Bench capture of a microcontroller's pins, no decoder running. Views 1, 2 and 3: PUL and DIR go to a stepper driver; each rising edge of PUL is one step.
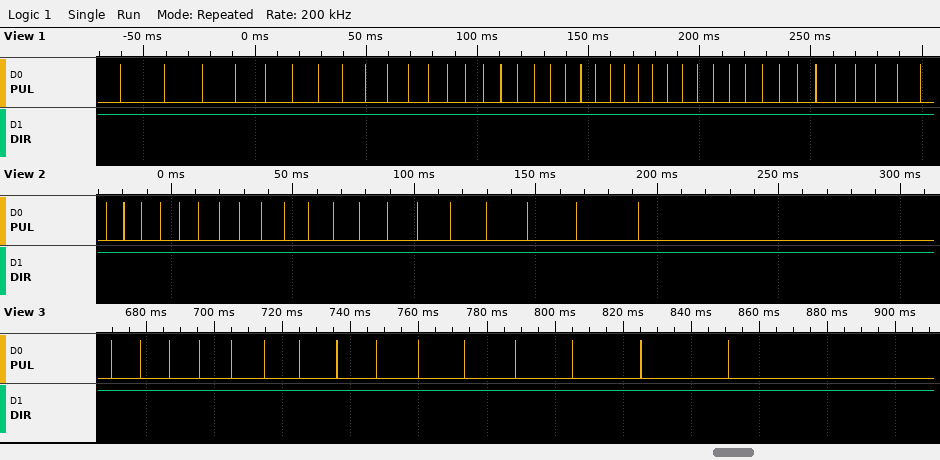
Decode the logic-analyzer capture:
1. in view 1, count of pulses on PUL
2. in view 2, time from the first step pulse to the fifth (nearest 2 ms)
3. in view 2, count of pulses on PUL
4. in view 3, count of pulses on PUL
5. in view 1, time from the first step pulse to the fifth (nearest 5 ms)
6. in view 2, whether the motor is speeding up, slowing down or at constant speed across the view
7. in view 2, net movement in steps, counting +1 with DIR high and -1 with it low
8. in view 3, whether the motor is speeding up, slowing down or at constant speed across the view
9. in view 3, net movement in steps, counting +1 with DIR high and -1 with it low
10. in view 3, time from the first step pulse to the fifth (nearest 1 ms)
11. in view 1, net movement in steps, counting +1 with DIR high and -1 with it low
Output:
41
30 ms
20
15
65 ms
slowing down
+20
slowing down
+15
35 ms
+41
